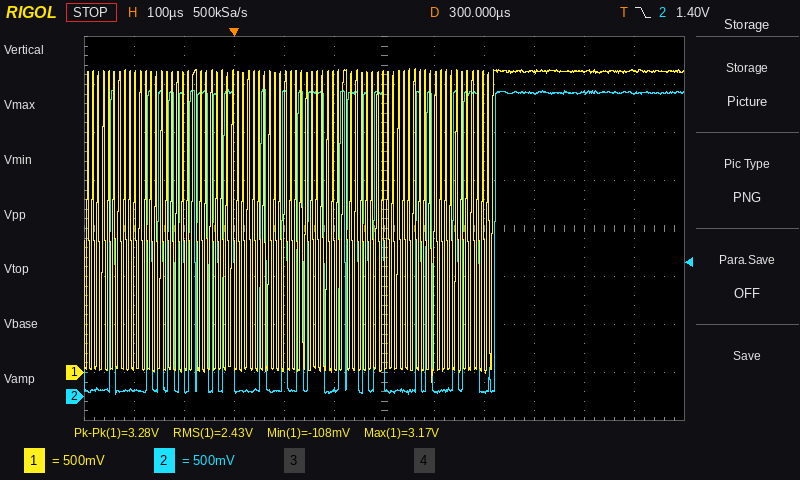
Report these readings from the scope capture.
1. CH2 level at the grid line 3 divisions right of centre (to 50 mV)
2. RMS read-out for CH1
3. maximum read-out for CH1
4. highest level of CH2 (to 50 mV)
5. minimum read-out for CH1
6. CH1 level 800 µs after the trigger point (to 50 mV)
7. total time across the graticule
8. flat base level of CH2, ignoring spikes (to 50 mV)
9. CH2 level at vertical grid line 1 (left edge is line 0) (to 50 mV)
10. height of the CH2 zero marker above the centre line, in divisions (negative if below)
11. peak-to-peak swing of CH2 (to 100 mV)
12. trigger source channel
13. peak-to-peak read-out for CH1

3.15 V
2.43 V
3.17 V
3.20 V
-108 mV
3.15 V
1.2 ms
50 mV
50 mV
-3.5 div
3.20 V
CH2
3.28 V
